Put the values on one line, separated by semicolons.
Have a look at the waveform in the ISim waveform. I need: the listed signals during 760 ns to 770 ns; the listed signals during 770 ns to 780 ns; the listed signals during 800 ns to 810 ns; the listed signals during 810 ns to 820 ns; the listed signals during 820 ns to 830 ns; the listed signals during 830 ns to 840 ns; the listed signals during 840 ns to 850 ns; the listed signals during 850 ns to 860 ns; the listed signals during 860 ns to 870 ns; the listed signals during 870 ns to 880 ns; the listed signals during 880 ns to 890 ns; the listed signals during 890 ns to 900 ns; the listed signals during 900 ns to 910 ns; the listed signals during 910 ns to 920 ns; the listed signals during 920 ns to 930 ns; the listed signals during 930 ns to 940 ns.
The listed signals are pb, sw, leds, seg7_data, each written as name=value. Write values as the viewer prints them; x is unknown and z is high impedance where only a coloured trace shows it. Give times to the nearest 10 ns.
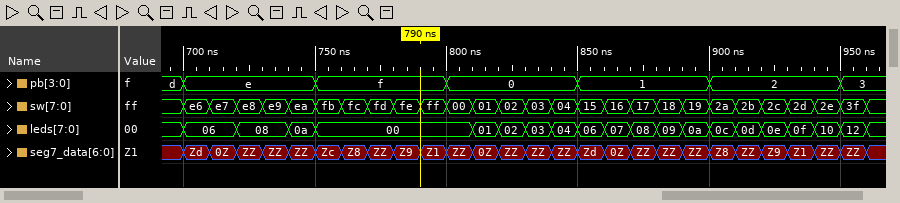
pb=f, sw=fc, leds=00, seg7_data=Z8; pb=f, sw=fd, leds=00, seg7_data=ZZ; pb=0, sw=00, leds=00, seg7_data=ZZ; pb=0, sw=01, leds=01, seg7_data=0Z; pb=0, sw=02, leds=02, seg7_data=ZZ; pb=0, sw=03, leds=03, seg7_data=ZZ; pb=0, sw=04, leds=04, seg7_data=ZZ; pb=1, sw=15, leds=06, seg7_data=Zd; pb=1, sw=16, leds=07, seg7_data=0Z; pb=1, sw=17, leds=08, seg7_data=ZZ; pb=1, sw=18, leds=09, seg7_data=ZZ; pb=1, sw=19, leds=0a, seg7_data=ZZ; pb=2, sw=2a, leds=0c, seg7_data=Z8; pb=2, sw=2b, leds=0d, seg7_data=ZZ; pb=2, sw=2c, leds=0e, seg7_data=Z9; pb=2, sw=2d, leds=0f, seg7_data=Z1
